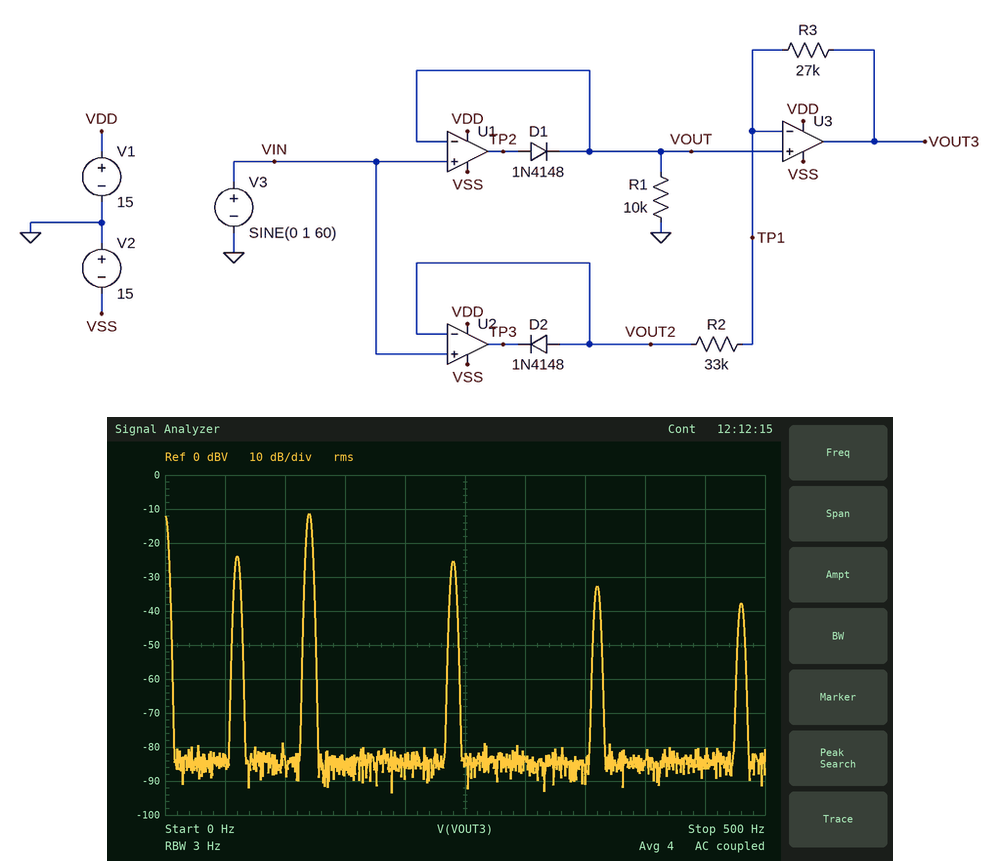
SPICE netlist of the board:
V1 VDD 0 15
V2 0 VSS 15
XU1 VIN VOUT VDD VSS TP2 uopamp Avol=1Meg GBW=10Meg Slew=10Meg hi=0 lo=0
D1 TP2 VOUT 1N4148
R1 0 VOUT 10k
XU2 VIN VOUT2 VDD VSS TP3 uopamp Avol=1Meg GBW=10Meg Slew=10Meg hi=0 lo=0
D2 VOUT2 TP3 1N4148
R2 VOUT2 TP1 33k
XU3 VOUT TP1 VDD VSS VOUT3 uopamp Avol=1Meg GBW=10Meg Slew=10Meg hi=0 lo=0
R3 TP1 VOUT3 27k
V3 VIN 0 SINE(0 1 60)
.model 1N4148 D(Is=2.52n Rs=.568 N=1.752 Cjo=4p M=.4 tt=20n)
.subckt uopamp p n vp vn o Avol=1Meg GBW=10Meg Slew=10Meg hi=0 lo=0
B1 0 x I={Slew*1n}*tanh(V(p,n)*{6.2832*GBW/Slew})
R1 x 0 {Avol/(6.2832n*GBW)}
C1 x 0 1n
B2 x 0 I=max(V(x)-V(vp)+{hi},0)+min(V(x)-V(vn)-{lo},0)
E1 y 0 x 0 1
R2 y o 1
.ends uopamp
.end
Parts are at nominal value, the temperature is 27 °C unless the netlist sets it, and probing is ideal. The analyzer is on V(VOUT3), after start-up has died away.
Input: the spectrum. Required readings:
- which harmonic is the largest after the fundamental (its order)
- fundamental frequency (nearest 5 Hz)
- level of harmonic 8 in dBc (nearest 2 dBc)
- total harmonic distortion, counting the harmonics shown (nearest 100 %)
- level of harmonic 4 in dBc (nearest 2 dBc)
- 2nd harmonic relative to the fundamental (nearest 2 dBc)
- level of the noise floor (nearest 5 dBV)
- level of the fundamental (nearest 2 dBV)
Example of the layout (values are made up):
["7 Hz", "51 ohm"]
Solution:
["2", "60 Hz", "-14 dBc", "400 %", "-2 dBc", "12 dBc", "-85 dBV", "-24 dBV"]
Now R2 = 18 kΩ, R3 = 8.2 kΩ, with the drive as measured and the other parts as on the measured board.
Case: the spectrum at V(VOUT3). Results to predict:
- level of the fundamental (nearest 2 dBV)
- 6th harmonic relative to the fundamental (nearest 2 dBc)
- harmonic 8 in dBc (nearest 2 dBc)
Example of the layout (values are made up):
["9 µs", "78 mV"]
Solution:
["-14 dBV", "-20 dBc", "-26 dBc"]
